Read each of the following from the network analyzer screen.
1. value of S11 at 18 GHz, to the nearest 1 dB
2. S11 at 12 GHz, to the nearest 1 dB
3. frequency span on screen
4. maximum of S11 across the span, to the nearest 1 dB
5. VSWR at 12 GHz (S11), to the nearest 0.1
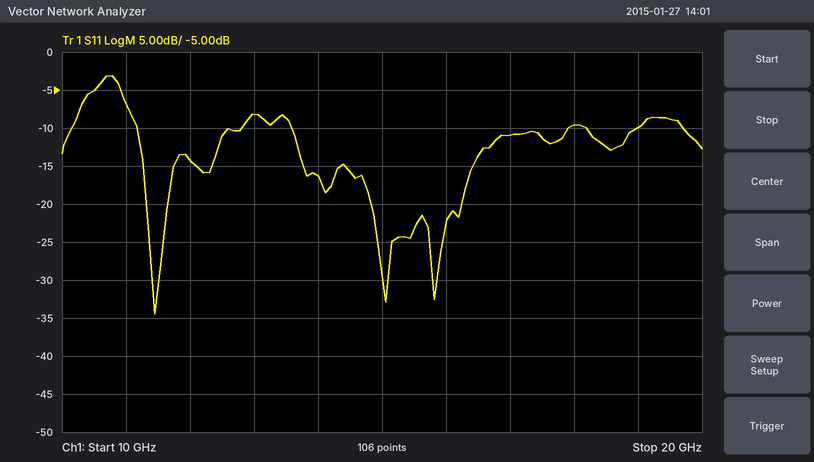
-10 dB
-14 dB
10 GHz
-3 dB
1.5
